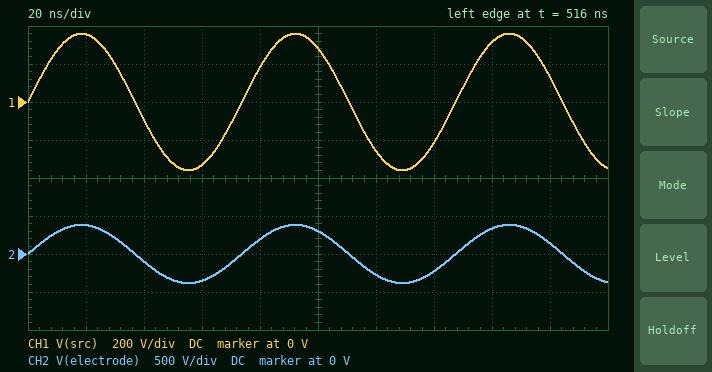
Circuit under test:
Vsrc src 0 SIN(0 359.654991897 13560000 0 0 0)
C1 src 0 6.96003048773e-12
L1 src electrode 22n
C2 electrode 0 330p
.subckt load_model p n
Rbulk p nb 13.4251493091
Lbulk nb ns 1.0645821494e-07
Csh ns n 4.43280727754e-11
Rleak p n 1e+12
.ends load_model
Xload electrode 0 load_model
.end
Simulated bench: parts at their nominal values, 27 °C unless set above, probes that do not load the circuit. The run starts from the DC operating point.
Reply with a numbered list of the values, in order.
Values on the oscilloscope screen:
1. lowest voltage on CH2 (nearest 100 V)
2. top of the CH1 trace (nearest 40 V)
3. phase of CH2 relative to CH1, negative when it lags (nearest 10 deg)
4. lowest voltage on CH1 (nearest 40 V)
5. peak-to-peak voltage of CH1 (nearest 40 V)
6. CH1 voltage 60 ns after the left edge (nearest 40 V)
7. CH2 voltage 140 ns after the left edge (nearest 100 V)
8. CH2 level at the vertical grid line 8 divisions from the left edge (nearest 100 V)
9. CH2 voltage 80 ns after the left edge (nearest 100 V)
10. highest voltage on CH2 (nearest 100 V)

1. -400 V
2. 360 V
3. 0 deg
4. -360 V
5. 720 V
6. -320 V
7. -200 V
8. 300 V
9. 200 V
10. 400 V
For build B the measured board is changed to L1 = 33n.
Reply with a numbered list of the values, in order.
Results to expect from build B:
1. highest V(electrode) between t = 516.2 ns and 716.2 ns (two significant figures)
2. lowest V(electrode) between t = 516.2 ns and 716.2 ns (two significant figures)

1. 400 V
2. -400 V
